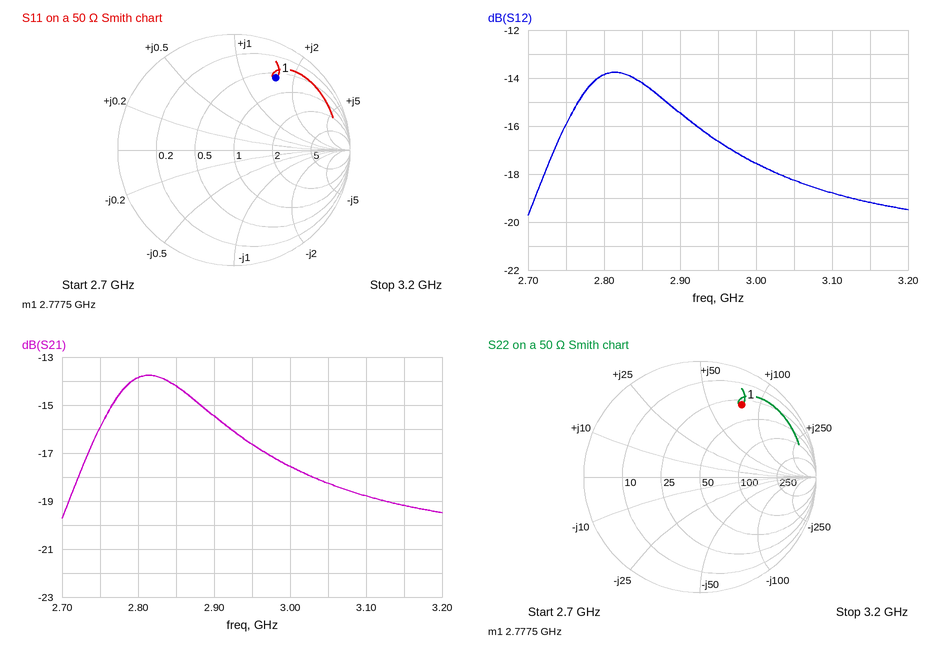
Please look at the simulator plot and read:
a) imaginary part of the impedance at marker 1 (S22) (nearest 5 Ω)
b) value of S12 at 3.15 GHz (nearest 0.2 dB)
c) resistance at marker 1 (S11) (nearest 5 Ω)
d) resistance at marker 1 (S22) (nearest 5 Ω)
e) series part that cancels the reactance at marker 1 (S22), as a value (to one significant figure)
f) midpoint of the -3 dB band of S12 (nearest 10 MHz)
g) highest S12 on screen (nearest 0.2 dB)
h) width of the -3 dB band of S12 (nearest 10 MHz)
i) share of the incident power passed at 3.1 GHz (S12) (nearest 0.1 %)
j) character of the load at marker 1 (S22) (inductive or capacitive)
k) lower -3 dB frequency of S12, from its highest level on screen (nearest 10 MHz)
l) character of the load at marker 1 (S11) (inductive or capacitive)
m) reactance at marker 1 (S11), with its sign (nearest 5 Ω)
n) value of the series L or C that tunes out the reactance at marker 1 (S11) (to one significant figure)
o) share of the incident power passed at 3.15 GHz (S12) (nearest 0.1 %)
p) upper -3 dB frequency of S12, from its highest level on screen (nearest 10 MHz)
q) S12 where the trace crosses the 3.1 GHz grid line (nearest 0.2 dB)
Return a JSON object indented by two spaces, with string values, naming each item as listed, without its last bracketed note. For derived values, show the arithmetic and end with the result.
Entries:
{
  "imaginary part of the impedance at marker 1 (S22)": "+80 Ω",
  "value of S12 at 3.15 GHz": "-19.2 dB",
  "resistance at marker 1 (S11)": "30 Ω",
  "resistance at marker 1 (S22)": "30 Ω",
  "series part that cancels the reactance at marker 1 (S22), as a value": "C = 1/(2π × 2.7775 GHz × 80 Ω) ≈ 716 fF, so 700 fF to one significant figure",
  "midpoint of the -3 dB band of S12": "2.85 GHz",
  "highest S12 on screen": "-13.8 dB",
  "width of the -3 dB band of S12": "2.96 GHz − 2.74 GHz = 220 MHz",
  "share of the incident power passed at 3.1 GHz (S12)": "10^(-18.8/10) ≈ 1.3 %",
  "character of the load at marker 1 (S22)": "inductive",
  "lower -3 dB frequency of S12, from its highest level on screen": "2.74 GHz",
  "character of the load at marker 1 (S11)": "inductive",
  "reactance at marker 1 (S11), with its sign": "+80 Ω",
  "value of the series L or C that tunes out the reactance at marker 1 (S11)": "C = 1/(2π × 2.7775 GHz × 80 Ω) ≈ 716 fF, so 700 fF to one significant figure",
  "share of the incident power passed at 3.15 GHz (S12)": "10^(-19.2/10) ≈ 1.2 %",
  "upper -3 dB frequency of S12, from its highest level on screen": "2.96 GHz",
  "S12 where the trace crosses the 3.1 GHz grid line": "-18.8 dB"
}
